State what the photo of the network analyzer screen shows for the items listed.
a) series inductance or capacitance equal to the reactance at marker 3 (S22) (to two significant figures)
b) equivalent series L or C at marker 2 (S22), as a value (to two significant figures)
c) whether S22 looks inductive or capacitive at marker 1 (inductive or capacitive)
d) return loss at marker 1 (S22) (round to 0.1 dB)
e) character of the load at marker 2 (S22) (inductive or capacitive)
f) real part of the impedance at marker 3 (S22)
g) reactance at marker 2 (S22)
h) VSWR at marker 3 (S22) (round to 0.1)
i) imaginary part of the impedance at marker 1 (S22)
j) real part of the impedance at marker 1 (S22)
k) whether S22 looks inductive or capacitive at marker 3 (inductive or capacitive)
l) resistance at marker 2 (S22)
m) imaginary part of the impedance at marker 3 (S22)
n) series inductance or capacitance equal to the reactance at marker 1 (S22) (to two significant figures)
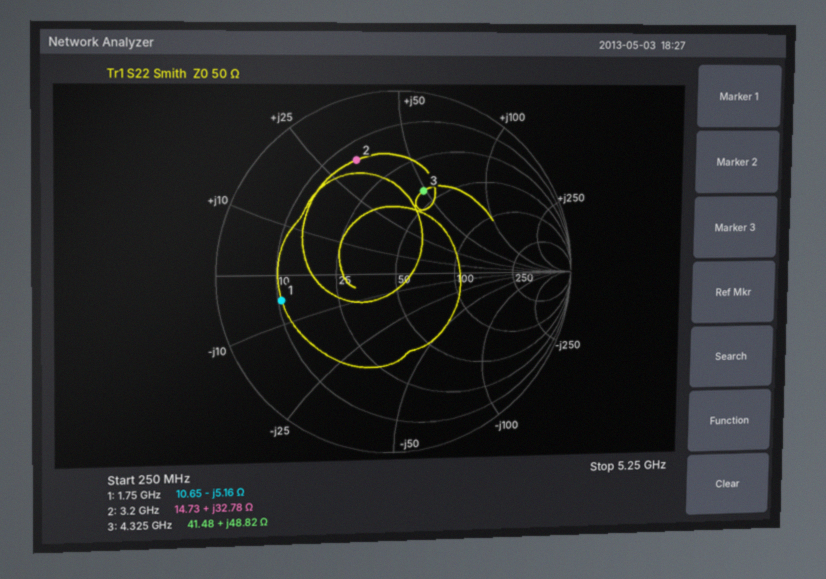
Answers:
1.8 nH
1.6 nH
capacitive
3.7 dB
inductive
41.48 Ω
+32.78 Ω
2.8
-5.16 Ω
10.65 Ω
inductive
14.73 Ω
+48.82 Ω
18 pF
